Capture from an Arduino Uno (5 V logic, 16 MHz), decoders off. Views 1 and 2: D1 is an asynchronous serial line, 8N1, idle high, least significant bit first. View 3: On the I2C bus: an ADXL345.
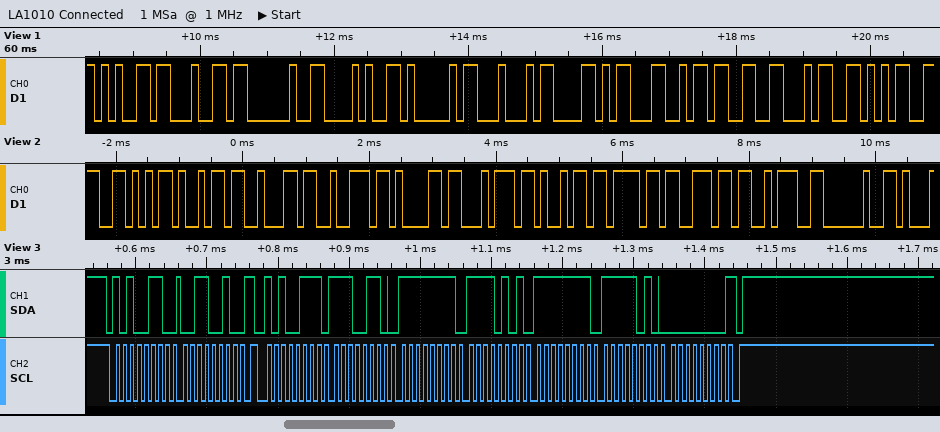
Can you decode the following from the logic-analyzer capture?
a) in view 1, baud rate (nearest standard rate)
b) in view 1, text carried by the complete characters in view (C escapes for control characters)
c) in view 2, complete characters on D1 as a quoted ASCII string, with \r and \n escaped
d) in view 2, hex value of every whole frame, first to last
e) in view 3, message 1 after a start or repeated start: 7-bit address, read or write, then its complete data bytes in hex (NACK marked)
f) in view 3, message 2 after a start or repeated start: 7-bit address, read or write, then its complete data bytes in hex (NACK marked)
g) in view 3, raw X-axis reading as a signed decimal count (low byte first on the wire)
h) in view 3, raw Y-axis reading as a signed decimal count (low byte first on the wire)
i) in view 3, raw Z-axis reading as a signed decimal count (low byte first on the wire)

9600 baud
"ed (ADXL345"
"Vibration: "
56 69 62 72 61 74 69 6F 6E 3A 20
0x53 write: 32
0x53 read: E6 FF F5 FF FA 00 NACK
-26
-11
250
